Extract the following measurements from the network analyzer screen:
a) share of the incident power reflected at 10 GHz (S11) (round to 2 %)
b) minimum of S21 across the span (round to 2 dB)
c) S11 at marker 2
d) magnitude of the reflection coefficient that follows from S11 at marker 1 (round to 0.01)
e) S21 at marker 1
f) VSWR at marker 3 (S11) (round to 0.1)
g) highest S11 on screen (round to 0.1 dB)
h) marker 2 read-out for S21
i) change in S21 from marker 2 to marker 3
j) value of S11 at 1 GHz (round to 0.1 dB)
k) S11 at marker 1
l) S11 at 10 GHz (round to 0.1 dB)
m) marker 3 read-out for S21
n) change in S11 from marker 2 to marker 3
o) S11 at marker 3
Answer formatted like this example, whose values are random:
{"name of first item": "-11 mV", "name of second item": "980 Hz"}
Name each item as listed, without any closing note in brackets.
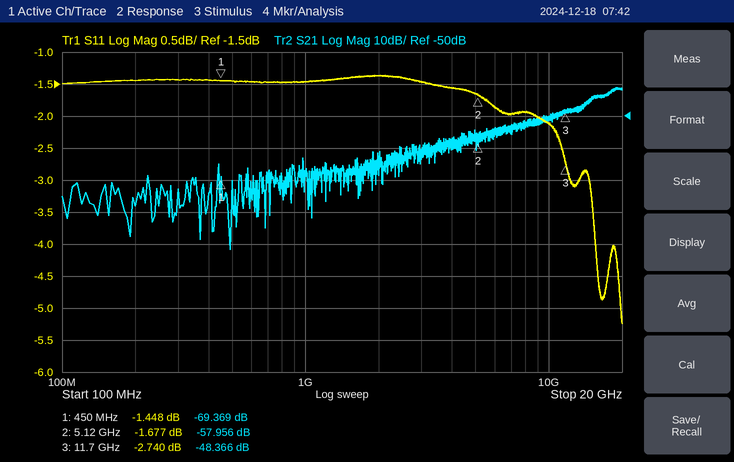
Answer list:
{"share of the incident power reflected at 10 GHz (S11)": "62 %", "minimum of S21 across the span": "-92 dB", "S11 at marker 2": "-1.677 dB", "magnitude of the reflection coefficient that follows from S11 at marker 1": "0.85", "S21 at marker 1": "-69.369 dB", "VSWR at marker 3 (S11)": "6.4", "highest S11 on screen": "-1.4 dB", "marker 2 read-out for S21": "-57.956 dB", "change in S21 from marker 2 to marker 3": "9.590 dB", "value of S11 at 1 GHz": "-1.5 dB", "S11 at marker 1": "-1.448 dB", "S11 at 10 GHz": "-2.1 dB", "marker 3 read-out for S21": "-48.366 dB", "change in S11 from marker 2 to marker 3": "-1.063 dB", "S11 at marker 3": "-2.740 dB"}
